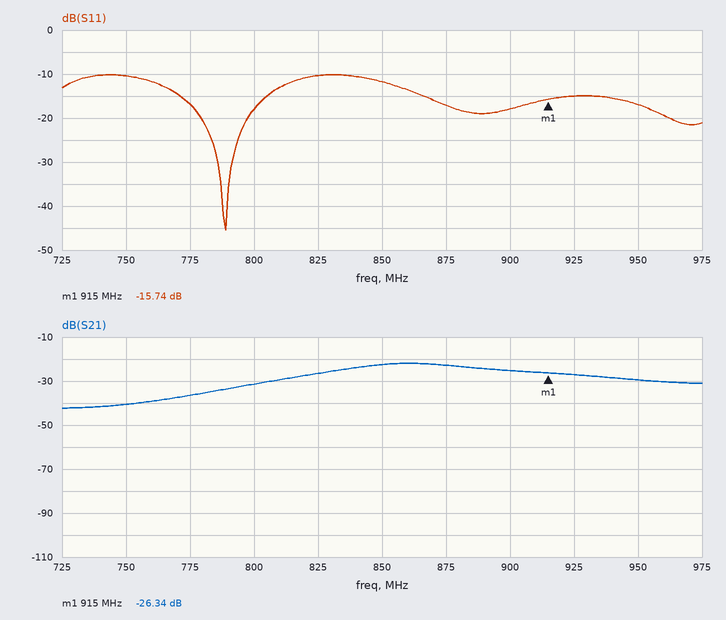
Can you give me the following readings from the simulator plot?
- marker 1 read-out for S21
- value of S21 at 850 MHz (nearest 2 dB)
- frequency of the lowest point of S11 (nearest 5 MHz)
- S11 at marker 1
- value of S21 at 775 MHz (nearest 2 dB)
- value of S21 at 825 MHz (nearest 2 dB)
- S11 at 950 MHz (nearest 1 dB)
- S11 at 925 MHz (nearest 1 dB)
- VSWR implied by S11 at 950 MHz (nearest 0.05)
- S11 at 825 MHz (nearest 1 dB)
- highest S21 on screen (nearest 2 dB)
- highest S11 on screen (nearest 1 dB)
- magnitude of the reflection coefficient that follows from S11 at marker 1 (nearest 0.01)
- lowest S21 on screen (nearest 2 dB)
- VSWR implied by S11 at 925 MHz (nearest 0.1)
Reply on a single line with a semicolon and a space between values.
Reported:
-26.34 dB; -22 dB; 790 MHz; -15.74 dB; -36 dB; -26 dB; -17 dB; -15 dB; 1.35; -10 dB; -22 dB; -10 dB; 0.16; -42 dB; 1.4
